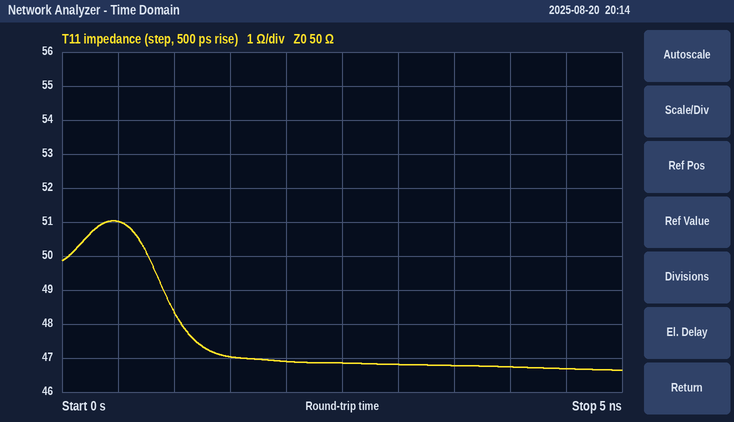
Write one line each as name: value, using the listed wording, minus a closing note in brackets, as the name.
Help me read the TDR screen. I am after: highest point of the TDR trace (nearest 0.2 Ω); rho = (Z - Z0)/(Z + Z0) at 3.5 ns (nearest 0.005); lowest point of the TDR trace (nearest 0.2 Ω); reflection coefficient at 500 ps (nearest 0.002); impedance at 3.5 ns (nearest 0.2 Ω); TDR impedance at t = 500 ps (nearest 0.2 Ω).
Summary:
highest point of the TDR trace: 51.0 Ω
rho = (Z - Z0)/(Z + Z0) at 3.5 ns: -0.035
lowest point of the TDR trace: 46.6 Ω
reflection coefficient at 500 ps: +0.010
impedance at 3.5 ns: 46.8 Ω
TDR impedance at t = 500 ps: 51.0 Ω
